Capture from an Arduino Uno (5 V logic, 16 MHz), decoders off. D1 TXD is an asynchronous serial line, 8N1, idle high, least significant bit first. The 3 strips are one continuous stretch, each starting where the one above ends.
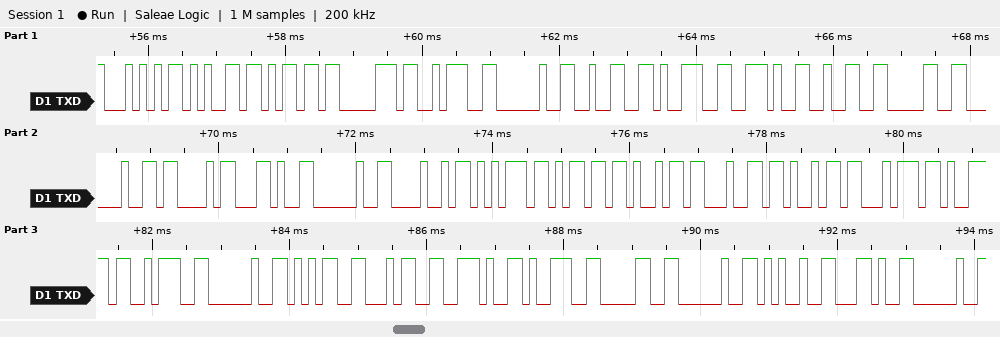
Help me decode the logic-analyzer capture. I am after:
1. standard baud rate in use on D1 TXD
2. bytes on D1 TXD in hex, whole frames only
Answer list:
9600 baud
54 65 6D 70 3A 20 32 39 2E 32 30 20 43 2C 20 48 75 6D 69 64 69 74 79 3A 20 35 34 2E 39 30 20 25 2C 20
